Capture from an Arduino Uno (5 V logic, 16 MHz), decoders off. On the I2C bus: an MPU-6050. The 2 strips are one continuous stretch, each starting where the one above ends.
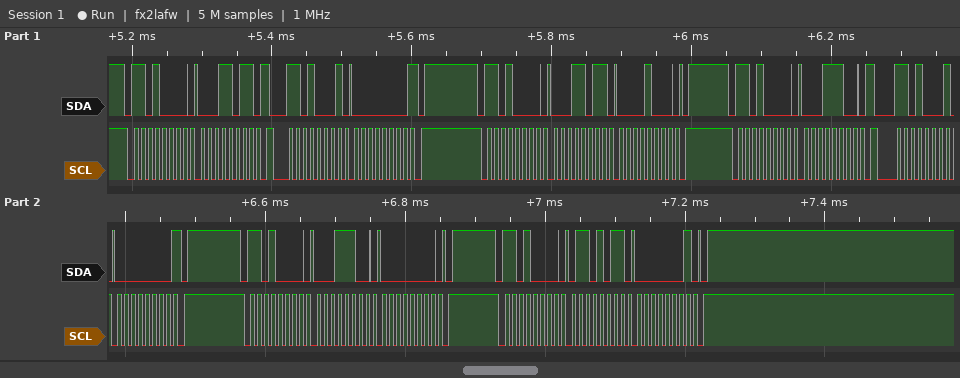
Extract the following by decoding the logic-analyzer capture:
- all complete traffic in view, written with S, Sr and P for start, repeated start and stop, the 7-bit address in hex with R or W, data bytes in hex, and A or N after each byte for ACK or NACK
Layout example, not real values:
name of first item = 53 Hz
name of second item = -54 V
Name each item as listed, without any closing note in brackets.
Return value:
all complete traffic in view, written with S, Sr and P for start, repeated start and stop, the 7-bit address in hex with R or W, data bytes in hex, and A or N after each byte for ACK or NACK = S 68W A 1B A Sr 68R A 00 N P S 68W A 1B A 08 A P S 68W A 1C A Sr 68R A 00 N P S 68W A 1C A 00 A P S 68W A 6B A 01 A P
